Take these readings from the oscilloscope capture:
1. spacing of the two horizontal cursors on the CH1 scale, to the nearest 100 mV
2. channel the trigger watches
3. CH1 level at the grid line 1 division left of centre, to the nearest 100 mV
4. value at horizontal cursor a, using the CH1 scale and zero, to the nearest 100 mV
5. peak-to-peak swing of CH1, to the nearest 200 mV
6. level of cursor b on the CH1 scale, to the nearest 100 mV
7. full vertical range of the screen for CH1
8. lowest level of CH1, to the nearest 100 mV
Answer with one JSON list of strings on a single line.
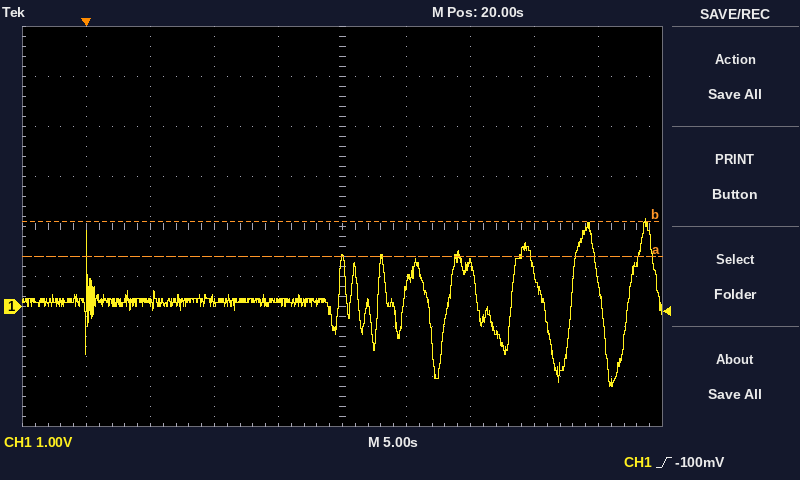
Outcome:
["700 mV", "CH1", "100 mV", "1.0 V", "3.4 V", "1.7 V", "8 V", "-1.6 V"]
